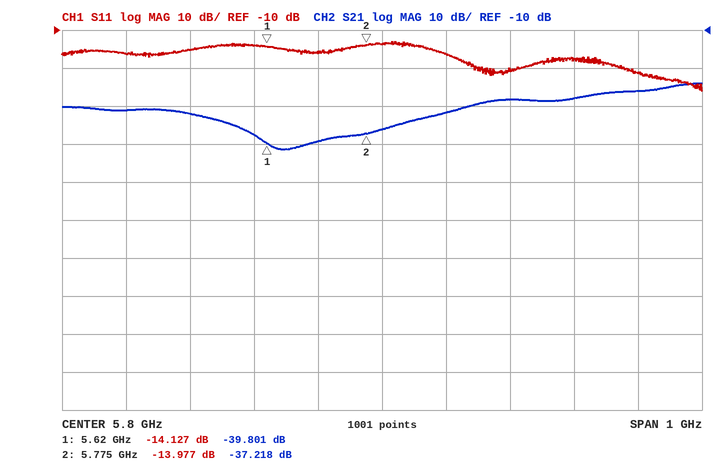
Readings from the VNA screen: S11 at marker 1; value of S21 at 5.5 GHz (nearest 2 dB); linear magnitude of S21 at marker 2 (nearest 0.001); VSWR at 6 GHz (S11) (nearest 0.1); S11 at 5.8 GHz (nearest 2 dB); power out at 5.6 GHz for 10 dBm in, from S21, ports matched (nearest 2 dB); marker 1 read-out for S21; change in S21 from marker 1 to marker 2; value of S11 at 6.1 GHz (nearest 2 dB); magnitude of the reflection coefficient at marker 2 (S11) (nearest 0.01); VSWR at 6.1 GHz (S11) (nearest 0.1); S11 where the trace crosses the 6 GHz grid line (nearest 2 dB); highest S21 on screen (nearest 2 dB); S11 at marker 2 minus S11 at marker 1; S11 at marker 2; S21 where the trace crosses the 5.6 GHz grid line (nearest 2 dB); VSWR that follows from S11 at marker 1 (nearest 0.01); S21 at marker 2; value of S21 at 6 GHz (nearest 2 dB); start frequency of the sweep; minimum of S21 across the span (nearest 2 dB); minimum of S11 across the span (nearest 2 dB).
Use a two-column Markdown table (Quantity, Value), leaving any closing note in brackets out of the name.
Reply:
| Quantity | Value |
|---|---|
| S11 at marker 1 | -14.127 dB |
| value of S21 at 5.5 GHz | -32 dB |
| linear magnitude of S21 at marker 2 | 0.014 |
| VSWR at 6 GHz (S11) | 1.2 |
| S11 at 5.8 GHz | -14 dB |
| power out at 5.6 GHz for 10 dBm in, from S21, ports matched | -28 dBm |
| marker 1 read-out for S21 | -39.801 dB |
| change in S21 from marker 1 to marker 2 | 2.583 dB |
| value of S11 at 6.1 GHz | -18 dB |
| magnitude of the reflection coefficient at marker 2 (S11) | 0.20 |
| VSWR at 6.1 GHz (S11) | 1.3 |
| S11 where the trace crosses the 6 GHz grid line | -20 dB |
| highest S21 on screen | -24 dB |
| S11 at marker 2 minus S11 at marker 1 | 0.150 dB |
| S11 at marker 2 | -13.977 dB |
| S21 where the trace crosses the 5.6 GHz grid line | -38 dB |
| VSWR that follows from S11 at marker 1 | 1.49 |
| S21 at marker 2 | -37.218 dB |
| value of S21 at 6 GHz | -28 dB |
| start frequency of the sweep | 5.3 GHz |
| minimum of S21 across the span | -42 dB |
| minimum of S11 across the span | -26 dB |
